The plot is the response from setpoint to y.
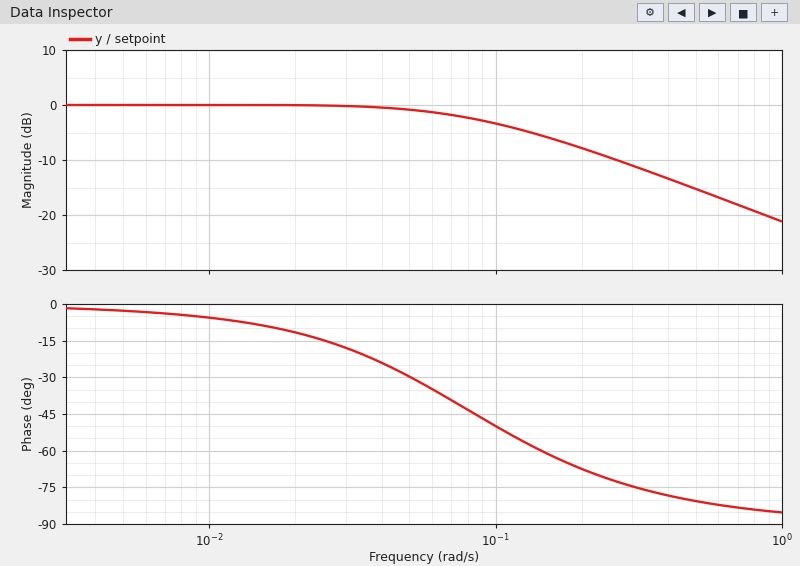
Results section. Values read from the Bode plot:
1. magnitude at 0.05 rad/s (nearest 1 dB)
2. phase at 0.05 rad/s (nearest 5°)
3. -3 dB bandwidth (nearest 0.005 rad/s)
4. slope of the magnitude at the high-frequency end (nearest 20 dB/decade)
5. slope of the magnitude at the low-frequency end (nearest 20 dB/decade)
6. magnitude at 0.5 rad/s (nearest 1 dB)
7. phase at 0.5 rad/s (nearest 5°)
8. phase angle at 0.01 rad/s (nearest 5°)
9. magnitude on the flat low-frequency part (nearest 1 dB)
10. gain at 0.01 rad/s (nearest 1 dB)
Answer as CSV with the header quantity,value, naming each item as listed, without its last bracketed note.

quantity,value
magnitude at 0.05 rad/s,-1 dB
phase at 0.05 rad/s,-30°
-3 dB bandwidth,0.095 rad/s
slope of the magnitude at the high-frequency end,-20 dB/decade
slope of the magnitude at the low-frequency end,0 dB/decade
magnitude at 0.5 rad/s,-15 dB
phase at 0.5 rad/s,-80°
phase angle at 0.01 rad/s,-5°
magnitude on the flat low-frequency part,0 dB
gain at 0.01 rad/s,0 dB
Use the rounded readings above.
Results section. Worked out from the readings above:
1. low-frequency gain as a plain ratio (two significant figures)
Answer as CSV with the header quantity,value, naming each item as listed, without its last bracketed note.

quantity,value
low-frequency gain as a plain ratio,1.0
